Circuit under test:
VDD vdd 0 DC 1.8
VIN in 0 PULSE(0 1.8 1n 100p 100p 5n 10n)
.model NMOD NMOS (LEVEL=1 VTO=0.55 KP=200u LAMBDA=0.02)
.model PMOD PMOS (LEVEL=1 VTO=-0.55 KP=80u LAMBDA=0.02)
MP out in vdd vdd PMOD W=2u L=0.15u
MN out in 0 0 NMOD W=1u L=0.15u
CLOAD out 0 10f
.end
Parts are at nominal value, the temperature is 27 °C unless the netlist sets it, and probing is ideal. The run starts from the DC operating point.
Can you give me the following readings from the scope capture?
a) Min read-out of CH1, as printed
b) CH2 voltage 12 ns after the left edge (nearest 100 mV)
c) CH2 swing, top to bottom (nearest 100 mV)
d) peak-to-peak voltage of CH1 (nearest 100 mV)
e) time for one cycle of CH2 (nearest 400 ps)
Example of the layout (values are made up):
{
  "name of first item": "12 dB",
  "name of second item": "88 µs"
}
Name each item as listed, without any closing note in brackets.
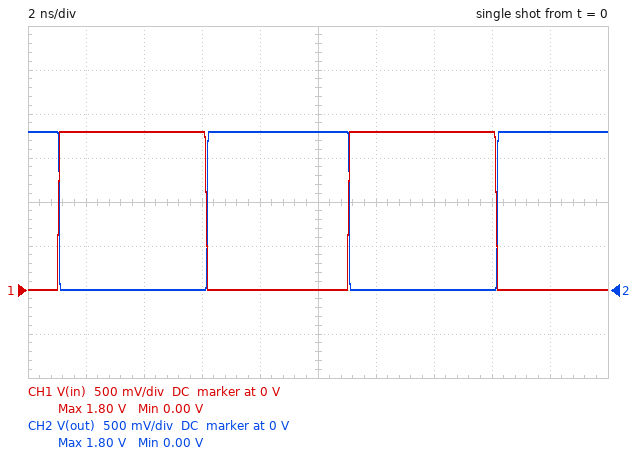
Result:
{
  "Min read-out of CH1, as printed": "0.00 V",
  "CH2 voltage 12 ns after the left edge": "0 V",
  "CH2 swing, top to bottom": "1.8 V",
  "peak-to-peak voltage of CH1": "1.8 V",
  "time for one cycle of CH2": "10.0 ns"
}
